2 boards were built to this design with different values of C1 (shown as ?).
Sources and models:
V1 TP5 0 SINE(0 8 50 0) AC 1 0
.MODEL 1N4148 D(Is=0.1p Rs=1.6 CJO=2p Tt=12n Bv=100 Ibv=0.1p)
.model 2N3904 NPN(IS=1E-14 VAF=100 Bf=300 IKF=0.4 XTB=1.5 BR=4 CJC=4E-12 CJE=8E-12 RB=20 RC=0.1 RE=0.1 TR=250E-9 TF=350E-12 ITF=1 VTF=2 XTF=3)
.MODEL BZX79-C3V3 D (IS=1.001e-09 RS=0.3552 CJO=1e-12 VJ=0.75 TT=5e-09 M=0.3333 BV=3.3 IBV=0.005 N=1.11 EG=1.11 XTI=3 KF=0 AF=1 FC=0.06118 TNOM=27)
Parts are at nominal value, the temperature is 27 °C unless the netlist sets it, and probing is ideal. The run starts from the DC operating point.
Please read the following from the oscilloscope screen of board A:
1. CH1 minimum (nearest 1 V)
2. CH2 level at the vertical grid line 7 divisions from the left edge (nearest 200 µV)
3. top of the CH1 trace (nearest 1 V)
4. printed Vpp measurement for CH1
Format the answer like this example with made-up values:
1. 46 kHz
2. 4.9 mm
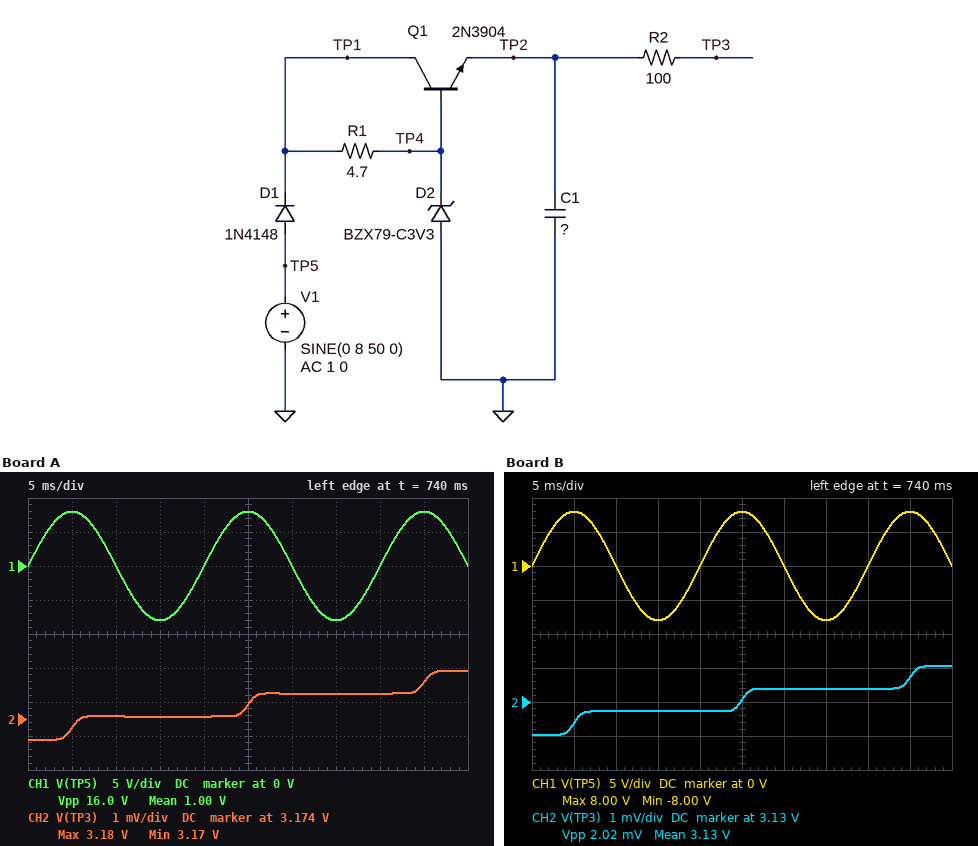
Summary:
1. -8 V
2. 3.1748 V
3. 8 V
4. 16.0 V
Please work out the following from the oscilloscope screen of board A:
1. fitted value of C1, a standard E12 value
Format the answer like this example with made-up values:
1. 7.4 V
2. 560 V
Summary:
1. 1.8 µF
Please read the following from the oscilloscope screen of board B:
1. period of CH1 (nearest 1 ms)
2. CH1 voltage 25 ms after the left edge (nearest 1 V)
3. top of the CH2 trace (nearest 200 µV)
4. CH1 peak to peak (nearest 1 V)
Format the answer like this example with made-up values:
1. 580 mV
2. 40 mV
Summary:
1. 20 ms
2. 8 V
3. 3.1310 V
4. 16 V
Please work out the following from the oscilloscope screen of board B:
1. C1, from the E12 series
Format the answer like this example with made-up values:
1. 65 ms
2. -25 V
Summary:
1. 10 µF
